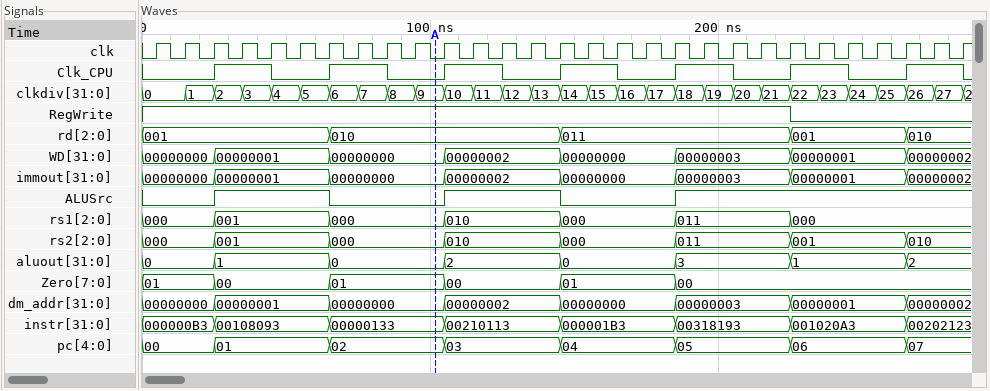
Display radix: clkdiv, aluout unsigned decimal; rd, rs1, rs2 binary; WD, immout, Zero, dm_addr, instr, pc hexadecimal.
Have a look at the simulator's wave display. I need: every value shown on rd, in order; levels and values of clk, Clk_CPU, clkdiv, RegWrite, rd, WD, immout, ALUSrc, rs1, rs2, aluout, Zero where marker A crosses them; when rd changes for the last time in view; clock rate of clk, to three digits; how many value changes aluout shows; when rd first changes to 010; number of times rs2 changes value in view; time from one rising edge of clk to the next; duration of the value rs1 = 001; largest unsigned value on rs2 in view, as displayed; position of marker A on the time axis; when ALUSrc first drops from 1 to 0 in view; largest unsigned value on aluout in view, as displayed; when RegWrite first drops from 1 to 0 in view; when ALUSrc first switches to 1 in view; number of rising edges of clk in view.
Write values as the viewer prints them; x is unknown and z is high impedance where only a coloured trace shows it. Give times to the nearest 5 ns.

001, 010, 011, 001, 010
clk=0, Clk_CPU=0, clkdiv=9, RegWrite=1, rd=010, WD=00000000, immout=00000000, ALUSrc=0, rs1=000, rs2=000, aluout=0, Zero=01
265 ns
100 MHz
7
65 ns
7
10 ns
40 ns
011
100 ns
65 ns
3
225 ns
25 ns
29
